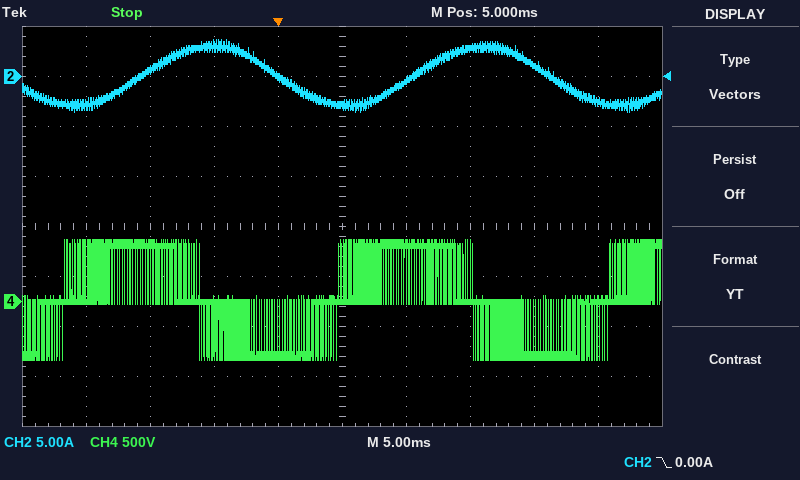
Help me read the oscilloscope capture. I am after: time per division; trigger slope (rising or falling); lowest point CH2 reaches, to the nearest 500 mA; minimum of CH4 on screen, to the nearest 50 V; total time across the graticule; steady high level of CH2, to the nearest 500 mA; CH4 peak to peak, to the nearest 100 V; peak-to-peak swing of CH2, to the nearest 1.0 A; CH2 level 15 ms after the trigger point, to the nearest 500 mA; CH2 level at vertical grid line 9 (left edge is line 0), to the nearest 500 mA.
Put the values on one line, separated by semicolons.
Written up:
5 ms; falling; -3.5 A; -600 V; 50 ms; 3.0 A; 1.20 kV; 7.0 A; 3.0 A; -2.5 A
